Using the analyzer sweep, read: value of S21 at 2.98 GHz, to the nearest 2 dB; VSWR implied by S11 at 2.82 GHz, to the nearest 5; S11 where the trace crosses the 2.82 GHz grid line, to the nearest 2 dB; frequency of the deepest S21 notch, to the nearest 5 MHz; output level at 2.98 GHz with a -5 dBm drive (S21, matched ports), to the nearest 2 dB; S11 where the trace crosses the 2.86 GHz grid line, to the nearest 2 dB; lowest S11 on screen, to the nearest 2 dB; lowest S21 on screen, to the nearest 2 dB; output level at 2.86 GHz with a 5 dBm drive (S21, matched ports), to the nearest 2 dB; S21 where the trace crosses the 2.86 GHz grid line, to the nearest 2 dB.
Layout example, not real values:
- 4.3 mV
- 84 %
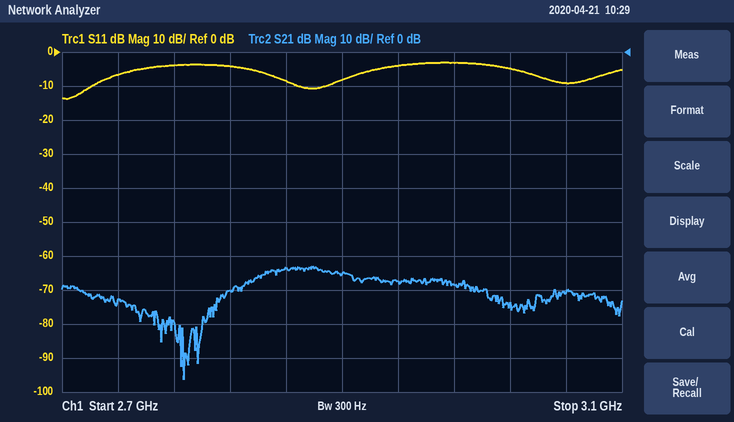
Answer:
- -68 dB
- 5
- -4 dB
- 2.785 GHz
- -74 dBm
- -8 dB
- -14 dB
- -96 dB
- -58 dBm
- -64 dB
